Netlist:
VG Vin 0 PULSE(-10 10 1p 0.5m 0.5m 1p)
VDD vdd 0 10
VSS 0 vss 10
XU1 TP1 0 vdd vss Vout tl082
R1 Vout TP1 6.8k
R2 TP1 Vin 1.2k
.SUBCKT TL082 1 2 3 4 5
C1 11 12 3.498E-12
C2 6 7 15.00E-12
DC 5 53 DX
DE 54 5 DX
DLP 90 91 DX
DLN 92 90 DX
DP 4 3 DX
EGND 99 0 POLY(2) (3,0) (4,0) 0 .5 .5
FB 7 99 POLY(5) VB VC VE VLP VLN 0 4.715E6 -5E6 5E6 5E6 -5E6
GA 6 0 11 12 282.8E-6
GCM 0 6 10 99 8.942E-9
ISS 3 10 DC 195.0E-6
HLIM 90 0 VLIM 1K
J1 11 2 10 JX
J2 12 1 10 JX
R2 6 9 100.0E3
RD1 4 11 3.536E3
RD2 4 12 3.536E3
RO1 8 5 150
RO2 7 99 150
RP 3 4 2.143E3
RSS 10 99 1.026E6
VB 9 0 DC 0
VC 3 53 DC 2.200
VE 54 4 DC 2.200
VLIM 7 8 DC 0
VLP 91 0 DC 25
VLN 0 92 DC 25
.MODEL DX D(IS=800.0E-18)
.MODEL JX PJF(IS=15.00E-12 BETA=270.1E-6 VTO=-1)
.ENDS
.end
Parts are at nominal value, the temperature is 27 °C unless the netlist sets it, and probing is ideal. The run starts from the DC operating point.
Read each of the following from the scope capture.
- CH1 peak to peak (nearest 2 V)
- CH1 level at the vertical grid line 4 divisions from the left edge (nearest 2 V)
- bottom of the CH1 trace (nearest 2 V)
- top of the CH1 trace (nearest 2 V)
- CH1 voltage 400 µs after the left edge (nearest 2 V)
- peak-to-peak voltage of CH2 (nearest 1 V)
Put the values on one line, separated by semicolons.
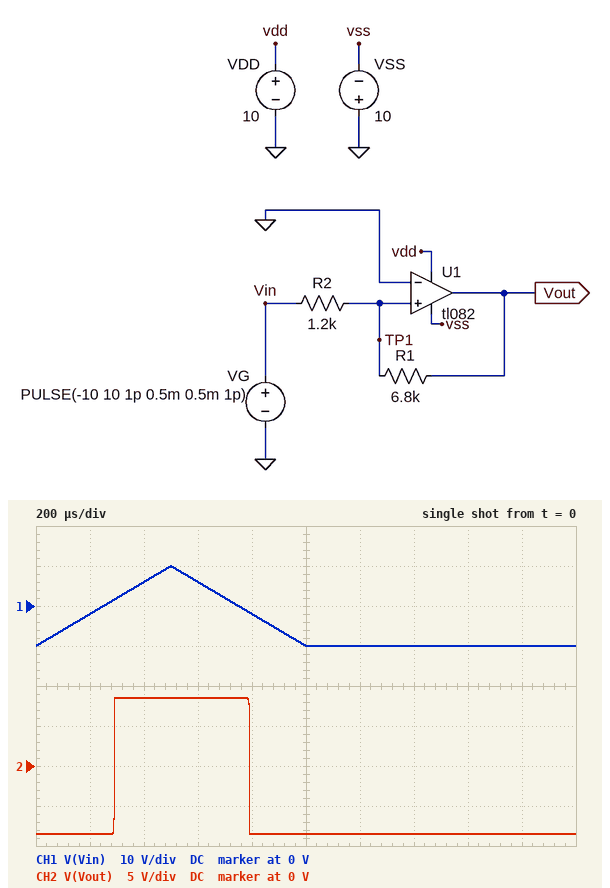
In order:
20 V; -2 V; -10 V; 10 V; 6 V; 17 V
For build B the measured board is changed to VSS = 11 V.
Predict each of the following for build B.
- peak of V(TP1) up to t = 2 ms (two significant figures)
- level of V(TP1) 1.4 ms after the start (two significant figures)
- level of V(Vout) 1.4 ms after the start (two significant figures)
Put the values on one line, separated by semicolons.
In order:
9.8 V; -9.9 V; -9.5 V
